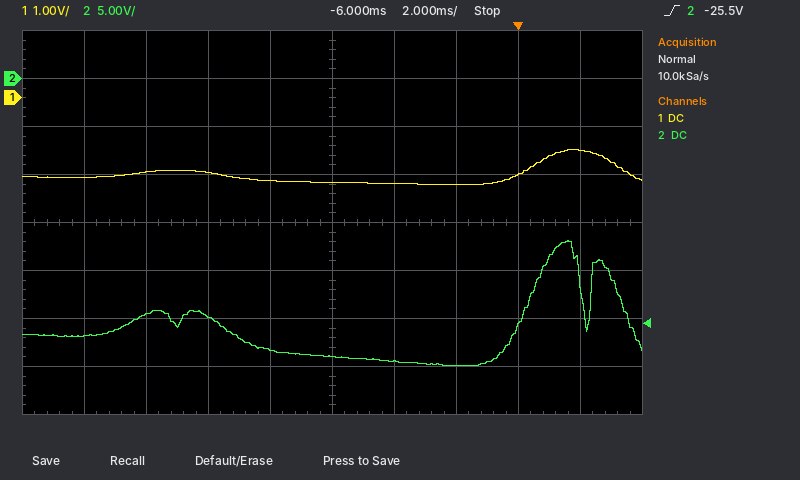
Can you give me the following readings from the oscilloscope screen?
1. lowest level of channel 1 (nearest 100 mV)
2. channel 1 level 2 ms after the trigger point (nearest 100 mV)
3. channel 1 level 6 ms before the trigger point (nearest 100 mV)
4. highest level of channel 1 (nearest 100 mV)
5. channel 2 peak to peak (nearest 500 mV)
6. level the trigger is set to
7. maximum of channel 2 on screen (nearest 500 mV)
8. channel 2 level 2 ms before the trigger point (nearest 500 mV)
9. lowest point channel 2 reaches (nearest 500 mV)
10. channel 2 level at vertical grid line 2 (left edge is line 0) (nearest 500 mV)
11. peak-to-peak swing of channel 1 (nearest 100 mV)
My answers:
-1.8 V
-1.1 V
-1.8 V
-1.1 V
13.0 V
-25.5 V
-17.0 V
-30.0 V
-30.0 V
-24.5 V
700 mV
